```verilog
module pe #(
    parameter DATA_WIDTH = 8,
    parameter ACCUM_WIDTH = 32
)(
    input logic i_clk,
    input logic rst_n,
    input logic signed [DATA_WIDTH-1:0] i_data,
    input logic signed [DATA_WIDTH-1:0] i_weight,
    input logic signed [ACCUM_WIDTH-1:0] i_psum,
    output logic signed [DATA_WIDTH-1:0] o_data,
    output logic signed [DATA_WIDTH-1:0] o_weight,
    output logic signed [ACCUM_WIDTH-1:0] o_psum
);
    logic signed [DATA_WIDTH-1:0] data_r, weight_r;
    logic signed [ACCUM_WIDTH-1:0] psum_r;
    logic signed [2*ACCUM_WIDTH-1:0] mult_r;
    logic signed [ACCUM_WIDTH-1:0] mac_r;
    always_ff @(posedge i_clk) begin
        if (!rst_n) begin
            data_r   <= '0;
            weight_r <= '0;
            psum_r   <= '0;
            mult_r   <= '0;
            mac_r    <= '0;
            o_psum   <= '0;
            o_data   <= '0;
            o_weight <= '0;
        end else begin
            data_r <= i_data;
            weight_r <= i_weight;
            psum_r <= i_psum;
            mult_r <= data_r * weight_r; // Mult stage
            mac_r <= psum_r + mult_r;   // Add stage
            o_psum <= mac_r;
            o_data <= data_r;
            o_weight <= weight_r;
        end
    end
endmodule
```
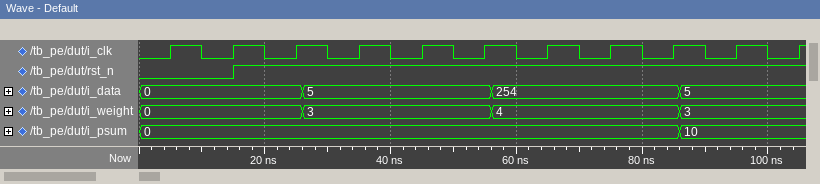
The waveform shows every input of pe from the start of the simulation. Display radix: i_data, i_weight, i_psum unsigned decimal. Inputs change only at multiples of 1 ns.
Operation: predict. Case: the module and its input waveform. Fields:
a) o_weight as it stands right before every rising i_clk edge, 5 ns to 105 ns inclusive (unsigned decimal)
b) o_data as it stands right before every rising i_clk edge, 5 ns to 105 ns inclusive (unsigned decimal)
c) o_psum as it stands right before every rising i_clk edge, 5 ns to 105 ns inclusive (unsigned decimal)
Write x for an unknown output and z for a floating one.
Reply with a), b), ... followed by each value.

a) x, 0, 0, 0, 0, 3, 3, 3, 4, 4, 4
b) x, 0, 0, 0, 0, 5, 5, 5, 254, 254, 254
c) x, 0, 0, 0, 0, 0, 0, 15, 15, 15, 4294967288
